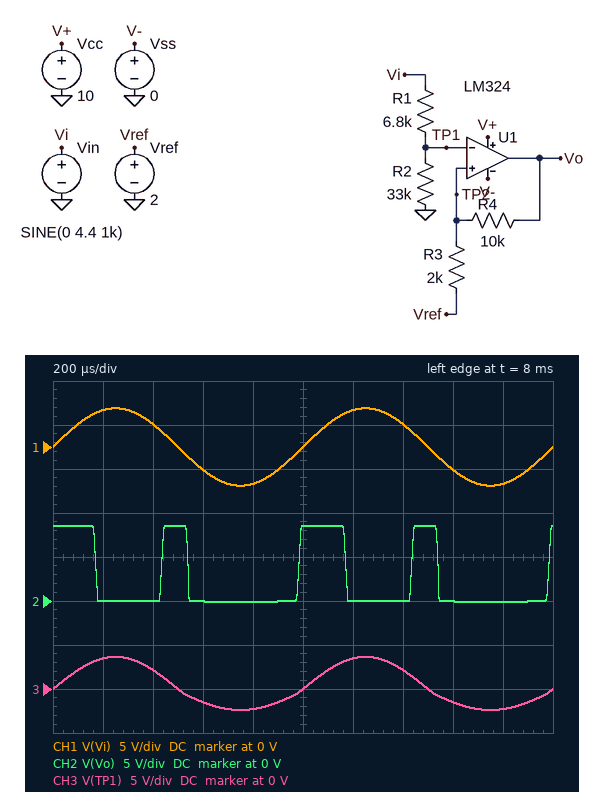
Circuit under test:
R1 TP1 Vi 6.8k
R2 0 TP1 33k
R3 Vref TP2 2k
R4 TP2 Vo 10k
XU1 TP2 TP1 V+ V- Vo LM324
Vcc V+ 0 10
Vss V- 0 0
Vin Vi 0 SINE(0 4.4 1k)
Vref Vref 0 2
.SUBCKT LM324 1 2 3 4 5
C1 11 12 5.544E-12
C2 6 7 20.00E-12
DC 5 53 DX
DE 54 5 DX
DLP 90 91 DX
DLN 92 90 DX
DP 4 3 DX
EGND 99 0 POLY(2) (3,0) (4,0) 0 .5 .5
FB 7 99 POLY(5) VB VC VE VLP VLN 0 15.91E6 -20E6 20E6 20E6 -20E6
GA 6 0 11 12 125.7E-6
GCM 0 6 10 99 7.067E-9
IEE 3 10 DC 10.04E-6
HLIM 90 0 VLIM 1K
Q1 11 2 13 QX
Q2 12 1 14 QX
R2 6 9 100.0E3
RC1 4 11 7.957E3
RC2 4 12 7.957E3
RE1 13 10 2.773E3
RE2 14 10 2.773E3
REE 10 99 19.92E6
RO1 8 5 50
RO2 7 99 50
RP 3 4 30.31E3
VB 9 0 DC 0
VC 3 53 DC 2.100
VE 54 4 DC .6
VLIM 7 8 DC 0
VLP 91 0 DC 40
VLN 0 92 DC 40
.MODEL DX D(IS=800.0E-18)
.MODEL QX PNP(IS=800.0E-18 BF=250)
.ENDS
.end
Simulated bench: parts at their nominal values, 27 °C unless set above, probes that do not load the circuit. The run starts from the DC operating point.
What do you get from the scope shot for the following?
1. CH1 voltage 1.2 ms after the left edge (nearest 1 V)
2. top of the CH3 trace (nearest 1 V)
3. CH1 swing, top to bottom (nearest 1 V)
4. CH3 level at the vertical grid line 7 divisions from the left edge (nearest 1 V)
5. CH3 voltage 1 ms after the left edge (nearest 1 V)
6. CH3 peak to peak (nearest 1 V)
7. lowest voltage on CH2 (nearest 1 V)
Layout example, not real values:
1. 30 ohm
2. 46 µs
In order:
1. 4 V
2. 4 V
3. 9 V
4. 2 V
5. 0 V
6. 6 V
7. 0 V
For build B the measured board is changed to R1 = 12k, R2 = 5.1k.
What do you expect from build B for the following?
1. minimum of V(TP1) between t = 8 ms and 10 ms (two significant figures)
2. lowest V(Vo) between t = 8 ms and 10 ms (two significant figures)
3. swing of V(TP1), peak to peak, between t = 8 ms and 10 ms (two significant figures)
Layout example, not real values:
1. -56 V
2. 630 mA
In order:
1. -1.1 V
2. -39 mV
3. 2.4 V
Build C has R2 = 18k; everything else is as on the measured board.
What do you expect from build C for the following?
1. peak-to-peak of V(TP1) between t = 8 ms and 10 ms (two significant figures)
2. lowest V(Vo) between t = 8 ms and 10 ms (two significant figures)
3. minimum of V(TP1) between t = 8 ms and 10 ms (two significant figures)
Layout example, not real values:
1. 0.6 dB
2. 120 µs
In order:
1. 5.4 V
2. -72 mV
3. -2.2 V
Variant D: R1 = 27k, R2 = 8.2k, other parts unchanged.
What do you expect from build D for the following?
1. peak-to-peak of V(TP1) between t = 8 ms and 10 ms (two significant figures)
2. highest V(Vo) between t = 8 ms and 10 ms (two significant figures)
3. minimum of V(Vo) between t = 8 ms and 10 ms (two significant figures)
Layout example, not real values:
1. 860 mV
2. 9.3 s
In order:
1. 1.8 V
2. 8.5 V
3. -17 mV
